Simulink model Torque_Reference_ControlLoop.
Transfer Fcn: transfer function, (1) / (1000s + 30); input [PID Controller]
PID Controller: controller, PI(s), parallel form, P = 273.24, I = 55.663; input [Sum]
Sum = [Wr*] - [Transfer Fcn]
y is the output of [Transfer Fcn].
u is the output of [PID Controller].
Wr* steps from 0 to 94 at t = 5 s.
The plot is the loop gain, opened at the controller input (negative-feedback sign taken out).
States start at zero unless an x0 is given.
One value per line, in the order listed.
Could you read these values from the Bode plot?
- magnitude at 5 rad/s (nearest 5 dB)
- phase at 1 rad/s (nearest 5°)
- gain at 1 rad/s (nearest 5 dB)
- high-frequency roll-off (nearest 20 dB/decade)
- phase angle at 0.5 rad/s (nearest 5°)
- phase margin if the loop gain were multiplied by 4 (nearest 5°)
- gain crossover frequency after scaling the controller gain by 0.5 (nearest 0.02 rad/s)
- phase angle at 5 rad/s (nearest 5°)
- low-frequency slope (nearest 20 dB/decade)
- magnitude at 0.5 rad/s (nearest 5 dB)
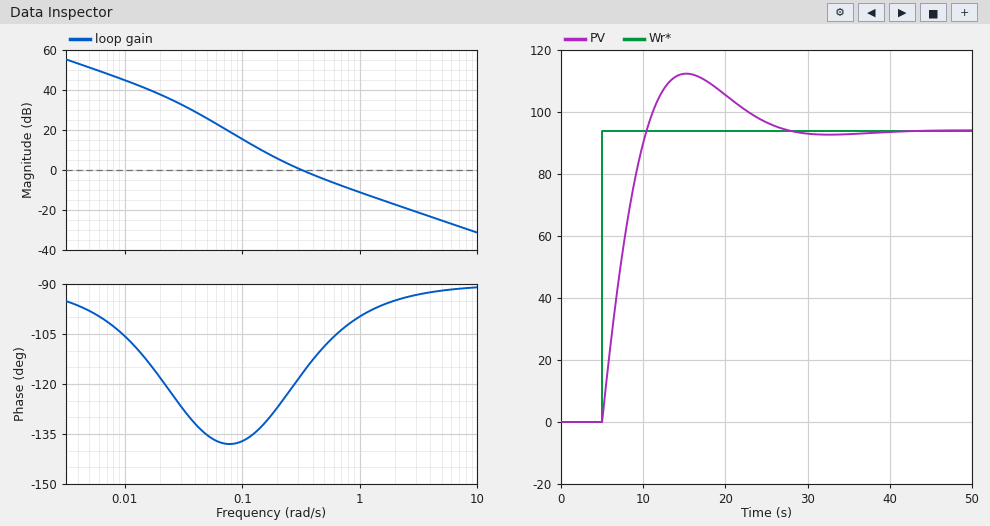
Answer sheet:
-25 dB
-100°
-10 dB
-20 dB/decade
-110°
80°
0.20 rad/s
-90°
-20 dB/decade
-5 dB
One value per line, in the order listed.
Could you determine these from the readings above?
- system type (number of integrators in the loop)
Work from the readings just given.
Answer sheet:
1
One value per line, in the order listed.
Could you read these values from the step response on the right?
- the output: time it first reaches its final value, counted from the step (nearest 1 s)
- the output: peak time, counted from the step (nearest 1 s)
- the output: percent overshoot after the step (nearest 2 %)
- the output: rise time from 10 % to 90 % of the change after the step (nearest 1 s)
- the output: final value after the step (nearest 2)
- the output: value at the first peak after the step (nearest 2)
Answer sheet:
5 s
10 s
20 %
4 s
94
112
